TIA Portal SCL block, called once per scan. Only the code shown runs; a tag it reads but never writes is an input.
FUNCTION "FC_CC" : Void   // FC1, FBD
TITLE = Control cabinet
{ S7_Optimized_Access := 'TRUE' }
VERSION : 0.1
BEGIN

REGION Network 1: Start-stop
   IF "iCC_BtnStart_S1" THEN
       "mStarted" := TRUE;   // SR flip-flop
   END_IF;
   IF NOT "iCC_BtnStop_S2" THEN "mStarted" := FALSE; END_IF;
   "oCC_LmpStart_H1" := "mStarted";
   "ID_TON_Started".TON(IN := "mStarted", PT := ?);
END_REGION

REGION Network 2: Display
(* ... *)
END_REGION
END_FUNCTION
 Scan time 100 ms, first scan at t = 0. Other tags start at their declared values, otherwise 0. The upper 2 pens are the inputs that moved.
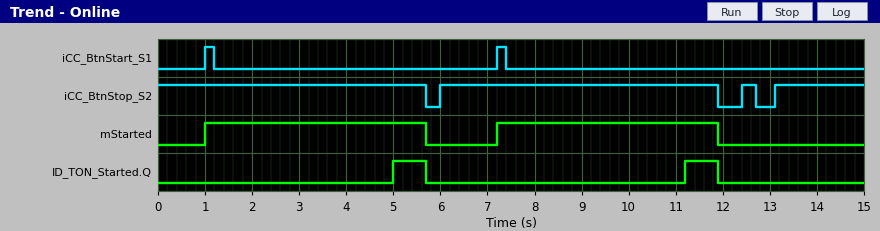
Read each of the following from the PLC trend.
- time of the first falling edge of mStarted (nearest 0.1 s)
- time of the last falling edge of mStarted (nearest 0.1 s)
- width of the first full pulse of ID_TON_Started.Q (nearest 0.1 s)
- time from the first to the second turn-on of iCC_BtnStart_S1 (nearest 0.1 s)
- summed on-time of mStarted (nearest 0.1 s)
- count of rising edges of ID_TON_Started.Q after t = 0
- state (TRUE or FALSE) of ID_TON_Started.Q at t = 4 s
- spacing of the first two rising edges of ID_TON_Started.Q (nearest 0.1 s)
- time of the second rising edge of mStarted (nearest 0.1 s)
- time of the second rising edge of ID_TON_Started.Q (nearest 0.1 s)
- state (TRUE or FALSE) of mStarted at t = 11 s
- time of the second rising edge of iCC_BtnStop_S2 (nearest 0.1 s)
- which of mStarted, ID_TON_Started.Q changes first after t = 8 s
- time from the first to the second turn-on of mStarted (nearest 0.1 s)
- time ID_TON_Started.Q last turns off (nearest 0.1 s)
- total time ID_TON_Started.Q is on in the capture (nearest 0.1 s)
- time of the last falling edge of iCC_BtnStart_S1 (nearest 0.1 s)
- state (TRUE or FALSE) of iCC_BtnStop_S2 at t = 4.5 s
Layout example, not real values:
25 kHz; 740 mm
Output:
5.7 s; 11.9 s; 0.7 s; 6.2 s; 9.4 s; 2; FALSE; 6.2 s; 7.2 s; 11.2 s; TRUE; 12.4 s; ID_TON_Started.Q; 6.2 s; 11.9 s; 1.4 s; 7.4 s; TRUE
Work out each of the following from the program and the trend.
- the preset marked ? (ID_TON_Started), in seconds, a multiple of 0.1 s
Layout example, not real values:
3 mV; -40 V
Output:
4.0 s
